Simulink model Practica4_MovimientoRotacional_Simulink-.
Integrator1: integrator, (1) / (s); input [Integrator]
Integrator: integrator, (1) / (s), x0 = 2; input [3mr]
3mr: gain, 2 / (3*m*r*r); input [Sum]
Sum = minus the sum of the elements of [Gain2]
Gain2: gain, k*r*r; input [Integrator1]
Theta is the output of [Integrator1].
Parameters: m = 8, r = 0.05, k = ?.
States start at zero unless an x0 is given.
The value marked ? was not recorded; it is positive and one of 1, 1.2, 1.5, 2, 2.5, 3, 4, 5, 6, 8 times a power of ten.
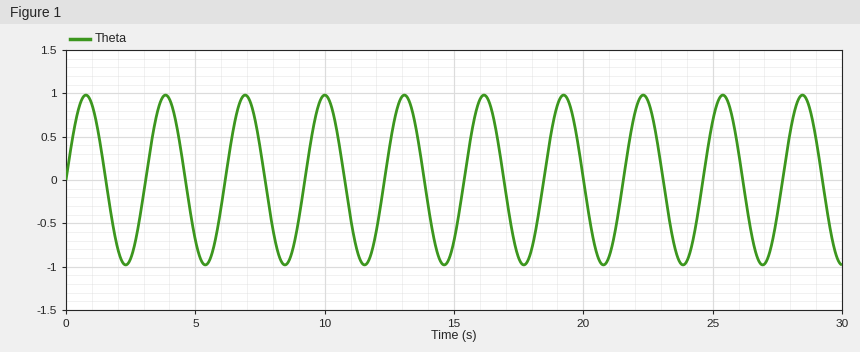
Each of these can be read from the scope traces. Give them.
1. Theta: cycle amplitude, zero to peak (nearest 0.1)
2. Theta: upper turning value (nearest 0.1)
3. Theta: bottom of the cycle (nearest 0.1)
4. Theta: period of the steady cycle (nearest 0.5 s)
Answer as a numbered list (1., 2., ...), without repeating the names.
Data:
1. 1.0
2. 1.0
3. -1.0
4. 3.0 s
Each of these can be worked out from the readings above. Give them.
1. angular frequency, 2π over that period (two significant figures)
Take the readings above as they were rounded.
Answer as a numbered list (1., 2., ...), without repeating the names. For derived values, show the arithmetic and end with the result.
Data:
1. 2π / 3 = 2.1 rad/s
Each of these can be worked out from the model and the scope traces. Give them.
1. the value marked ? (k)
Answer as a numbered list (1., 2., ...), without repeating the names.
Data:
1. 50
